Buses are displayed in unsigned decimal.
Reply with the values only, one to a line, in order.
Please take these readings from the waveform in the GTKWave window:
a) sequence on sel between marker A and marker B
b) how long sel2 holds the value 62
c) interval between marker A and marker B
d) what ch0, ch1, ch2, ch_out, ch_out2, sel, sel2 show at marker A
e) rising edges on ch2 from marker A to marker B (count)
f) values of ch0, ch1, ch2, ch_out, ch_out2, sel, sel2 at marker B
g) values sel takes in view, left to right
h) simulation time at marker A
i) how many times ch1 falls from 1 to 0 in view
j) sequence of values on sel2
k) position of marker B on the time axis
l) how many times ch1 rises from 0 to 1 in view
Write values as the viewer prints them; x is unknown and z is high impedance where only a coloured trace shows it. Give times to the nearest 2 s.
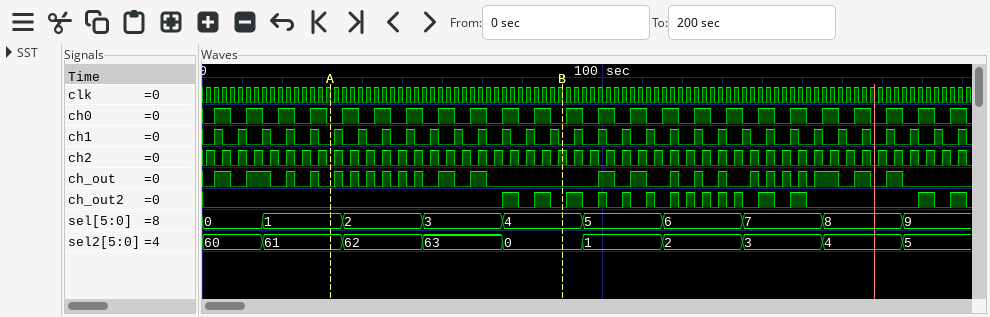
1, 2, 3, 4
20 s
58 s
ch0=0, ch1=0, ch2=0, ch_out=0, ch_out2=0, sel=1, sel2=61
15
ch0=0, ch1=0, ch2=1, ch_out=0, ch_out2=0, sel=4, sel2=0
0, 1, 2, 3, 4, 5, 6, 7, 8, 9
32 s
32
60, 61, 62, 63, 0, 1, 2, 3, 4, 5
90 s
32
